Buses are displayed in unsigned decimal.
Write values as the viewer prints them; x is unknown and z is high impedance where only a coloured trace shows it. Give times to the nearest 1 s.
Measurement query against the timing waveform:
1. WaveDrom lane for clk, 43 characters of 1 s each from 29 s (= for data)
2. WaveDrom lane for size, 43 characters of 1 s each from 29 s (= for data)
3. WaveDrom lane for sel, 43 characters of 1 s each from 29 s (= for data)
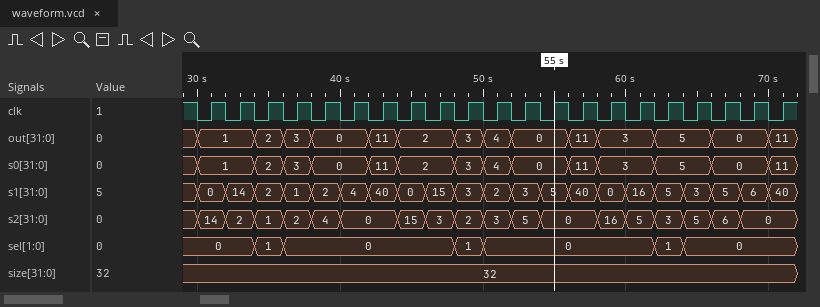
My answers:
{name: 'clk', wave: '1010101010101010101010101010101010101010101'}
{name: 'size', wave: '=..........................................', data: '32'}
{name: 'sel', wave: '=....=.=...........=.=...........=.=.......', data: '0 1 0 1 0 1 0'}
